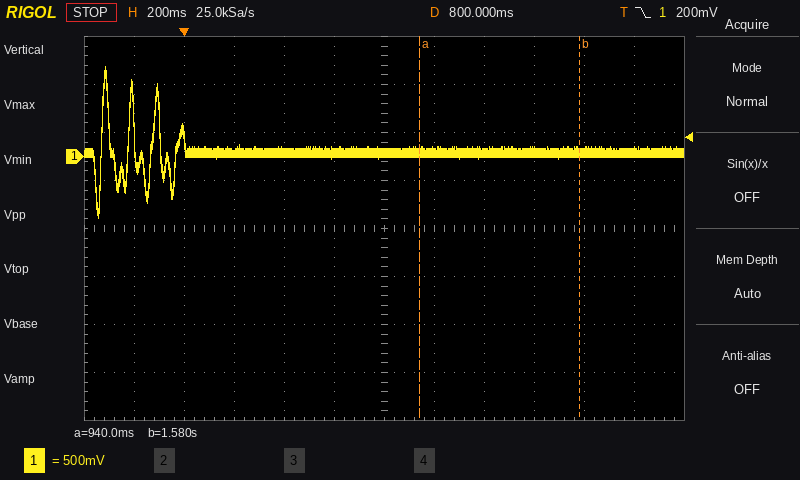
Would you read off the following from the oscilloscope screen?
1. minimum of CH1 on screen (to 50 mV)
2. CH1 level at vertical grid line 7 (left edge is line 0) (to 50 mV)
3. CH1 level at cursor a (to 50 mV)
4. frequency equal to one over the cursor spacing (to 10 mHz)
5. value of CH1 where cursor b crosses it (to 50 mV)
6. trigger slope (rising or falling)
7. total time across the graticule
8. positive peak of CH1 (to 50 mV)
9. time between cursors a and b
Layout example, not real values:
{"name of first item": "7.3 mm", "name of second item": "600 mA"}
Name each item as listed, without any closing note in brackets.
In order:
{"minimum of CH1 on screen": "-650 mV", "CH1 level at vertical grid line 7 (left edge is line 0)": "50 mV", "CH1 level at cursor a": "50 mV", "frequency equal to one over the cursor spacing": "1.56 Hz", "value of CH1 where cursor b crosses it": "50 mV", "trigger slope": "falling", "total time across the graticule": "2.4 s", "positive peak of CH1": "950 mV", "time between cursors a and b": "640 ms"}
